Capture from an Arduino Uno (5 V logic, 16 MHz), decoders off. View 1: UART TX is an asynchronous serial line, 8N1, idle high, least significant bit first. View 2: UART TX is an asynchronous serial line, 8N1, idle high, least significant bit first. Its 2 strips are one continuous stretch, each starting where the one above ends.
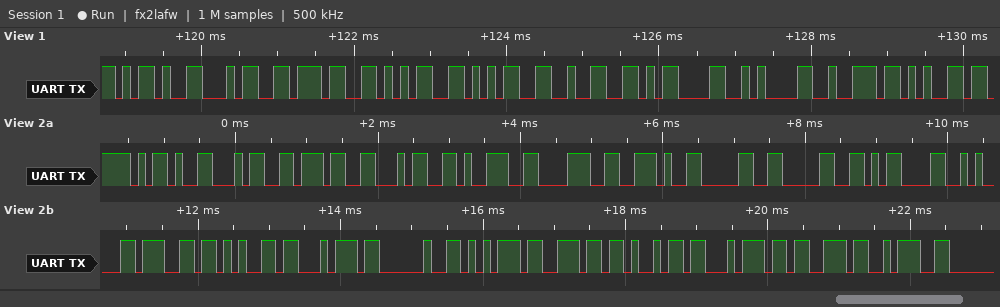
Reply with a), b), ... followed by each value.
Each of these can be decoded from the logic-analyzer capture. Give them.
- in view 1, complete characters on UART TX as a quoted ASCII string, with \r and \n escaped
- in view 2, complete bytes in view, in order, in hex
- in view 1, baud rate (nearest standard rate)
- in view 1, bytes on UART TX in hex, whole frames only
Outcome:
a) "-47552\r\nre"
b) 2D 34 37 34 39 38 2E 30 30 0D 0A 67 65 74 20 75 6E 69 74 73 3A
c) 9600 baud
d) 2D 34 37 35 35 32 0D 0A 72 65
